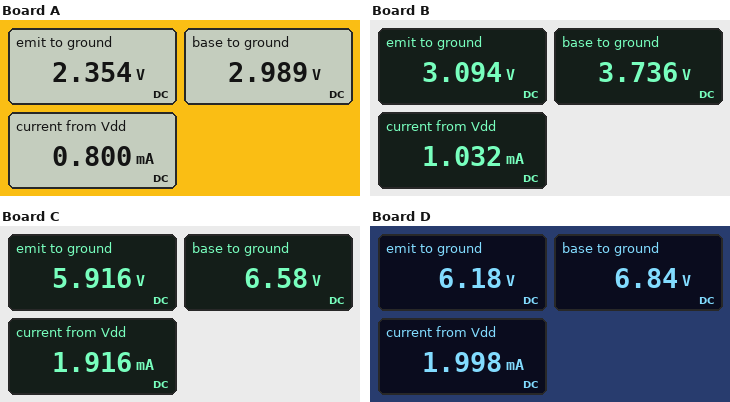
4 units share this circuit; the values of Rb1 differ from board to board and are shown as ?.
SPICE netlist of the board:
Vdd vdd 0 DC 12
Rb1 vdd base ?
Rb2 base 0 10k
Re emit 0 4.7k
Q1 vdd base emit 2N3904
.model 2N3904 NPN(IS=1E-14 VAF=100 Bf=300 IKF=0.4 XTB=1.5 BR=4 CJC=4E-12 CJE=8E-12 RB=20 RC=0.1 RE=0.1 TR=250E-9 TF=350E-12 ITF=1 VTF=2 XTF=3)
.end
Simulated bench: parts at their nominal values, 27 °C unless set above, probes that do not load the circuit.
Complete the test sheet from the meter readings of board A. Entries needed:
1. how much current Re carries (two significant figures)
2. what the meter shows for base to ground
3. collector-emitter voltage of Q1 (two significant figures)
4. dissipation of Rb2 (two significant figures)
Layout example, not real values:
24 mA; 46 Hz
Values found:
500 µA; 2.989 V; 9.6 V; 890 µW
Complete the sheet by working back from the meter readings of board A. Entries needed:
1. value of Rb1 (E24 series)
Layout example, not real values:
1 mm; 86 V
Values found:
30 kΩ
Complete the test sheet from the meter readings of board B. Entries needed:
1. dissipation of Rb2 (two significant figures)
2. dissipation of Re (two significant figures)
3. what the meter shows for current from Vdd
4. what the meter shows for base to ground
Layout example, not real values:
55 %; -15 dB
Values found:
1.4 mW; 2.0 mW; 1.032 mA; 3.736 V
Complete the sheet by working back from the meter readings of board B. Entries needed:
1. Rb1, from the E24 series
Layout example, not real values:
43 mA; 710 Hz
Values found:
22 kΩ
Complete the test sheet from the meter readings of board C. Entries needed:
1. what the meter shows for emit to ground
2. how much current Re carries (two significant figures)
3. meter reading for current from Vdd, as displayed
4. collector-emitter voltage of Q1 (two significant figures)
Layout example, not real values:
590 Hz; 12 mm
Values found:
5.916 V; 1.3 mA; 1.916 mA; 6.1 V
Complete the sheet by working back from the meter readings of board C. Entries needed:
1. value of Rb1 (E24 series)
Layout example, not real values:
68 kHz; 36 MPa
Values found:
8.2 kΩ
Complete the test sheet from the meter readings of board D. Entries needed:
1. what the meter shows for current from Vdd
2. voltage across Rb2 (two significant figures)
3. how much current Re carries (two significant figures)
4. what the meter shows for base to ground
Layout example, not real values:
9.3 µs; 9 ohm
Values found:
1.998 mA; 6.8 V; 1.3 mA; 6.84 V
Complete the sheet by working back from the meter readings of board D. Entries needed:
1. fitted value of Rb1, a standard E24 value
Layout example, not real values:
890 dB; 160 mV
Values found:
7.5 kΩ
